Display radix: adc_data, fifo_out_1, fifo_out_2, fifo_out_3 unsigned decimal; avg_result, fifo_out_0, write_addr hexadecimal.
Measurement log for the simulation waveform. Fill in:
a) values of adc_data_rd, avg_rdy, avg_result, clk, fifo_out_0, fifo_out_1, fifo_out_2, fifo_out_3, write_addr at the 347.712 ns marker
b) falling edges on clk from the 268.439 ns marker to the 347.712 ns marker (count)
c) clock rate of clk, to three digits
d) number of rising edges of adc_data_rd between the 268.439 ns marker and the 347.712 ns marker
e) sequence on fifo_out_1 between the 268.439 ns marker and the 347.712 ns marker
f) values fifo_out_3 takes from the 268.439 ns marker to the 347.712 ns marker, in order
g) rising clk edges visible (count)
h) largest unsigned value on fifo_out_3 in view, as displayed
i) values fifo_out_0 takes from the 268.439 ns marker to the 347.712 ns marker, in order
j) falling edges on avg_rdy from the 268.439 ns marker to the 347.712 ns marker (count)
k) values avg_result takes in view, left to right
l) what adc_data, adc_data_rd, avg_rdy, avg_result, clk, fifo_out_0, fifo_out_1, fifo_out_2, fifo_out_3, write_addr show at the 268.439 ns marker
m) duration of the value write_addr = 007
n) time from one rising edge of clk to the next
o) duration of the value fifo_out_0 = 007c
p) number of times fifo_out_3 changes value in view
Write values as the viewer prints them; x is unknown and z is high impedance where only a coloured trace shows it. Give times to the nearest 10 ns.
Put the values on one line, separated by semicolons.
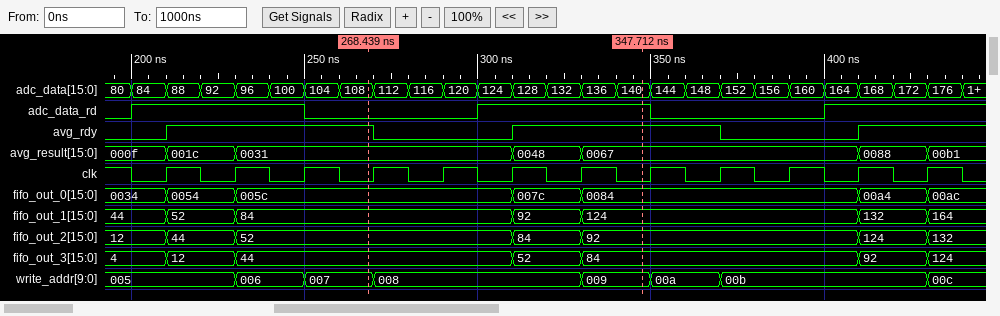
adc_data_rd=1, avg_rdy=1, avg_result=0067, clk=0, fifo_out_0=0084, fifo_out_1=124, fifo_out_2=92, fifo_out_3=84, write_addr=009; 4; 50.0 MHz; 1; 84, 92, 124; 44, 52, 84; 12; 124; 005c, 007c, 0084; 1; 000f, 001c, 0031, 0048, 0067, 0088, 00b1; adc_data=108, adc_data_rd=0, avg_rdy=1, avg_result=0031, clk=0, fifo_out_0=005c, fifo_out_1=84, fifo_out_2=52, fifo_out_3=44, write_addr=007; 20 ns; 20 ns; 20 ns; 6
